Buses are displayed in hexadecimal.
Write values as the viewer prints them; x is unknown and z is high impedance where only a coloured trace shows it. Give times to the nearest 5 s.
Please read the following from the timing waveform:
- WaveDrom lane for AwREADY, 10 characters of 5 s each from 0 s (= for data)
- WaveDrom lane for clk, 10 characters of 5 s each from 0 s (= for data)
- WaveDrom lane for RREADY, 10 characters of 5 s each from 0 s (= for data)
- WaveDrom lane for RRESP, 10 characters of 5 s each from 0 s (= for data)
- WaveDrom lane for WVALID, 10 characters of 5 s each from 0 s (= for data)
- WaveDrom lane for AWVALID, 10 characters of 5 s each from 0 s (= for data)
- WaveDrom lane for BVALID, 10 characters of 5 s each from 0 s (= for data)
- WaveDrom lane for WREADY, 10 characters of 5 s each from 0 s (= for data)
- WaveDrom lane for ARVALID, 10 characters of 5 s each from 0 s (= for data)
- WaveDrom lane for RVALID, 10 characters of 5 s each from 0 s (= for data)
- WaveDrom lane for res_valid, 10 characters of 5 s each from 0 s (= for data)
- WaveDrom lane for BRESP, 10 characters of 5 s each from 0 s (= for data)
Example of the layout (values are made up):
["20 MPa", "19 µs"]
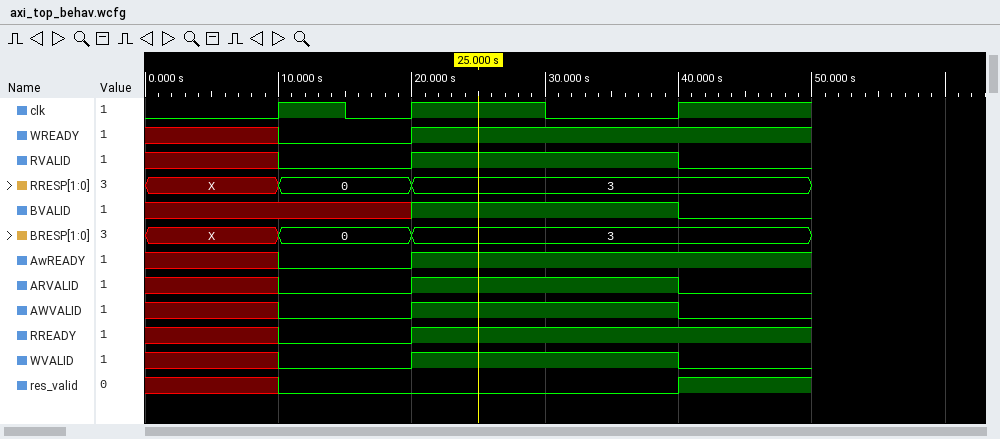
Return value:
["{name: 'AwREADY', wave: 'x.0.1.....'}", "{name: 'clk', wave: '0.101.0.1.'}", "{name: 'RREADY', wave: 'x.0.1.....'}", "{name: 'RRESP', wave: 'x.=.=.....', data: '0 3'}", "{name: 'WVALID', wave: 'x.0.1...0.'}", "{name: 'AWVALID', wave: 'x.0.1...0.'}", "{name: 'BVALID', wave: 'x...1...0.'}", "{name: 'WREADY', wave: 'x.0.1.....'}", "{name: 'ARVALID', wave: 'x.0.1...0.'}", "{name: 'RVALID', wave: 'x.0.1...0.'}", "{name: 'res_valid', wave: 'x.0.....1.'}", "{name: 'BRESP', wave: 'x.=.=.....', data: '0 3'}"]
